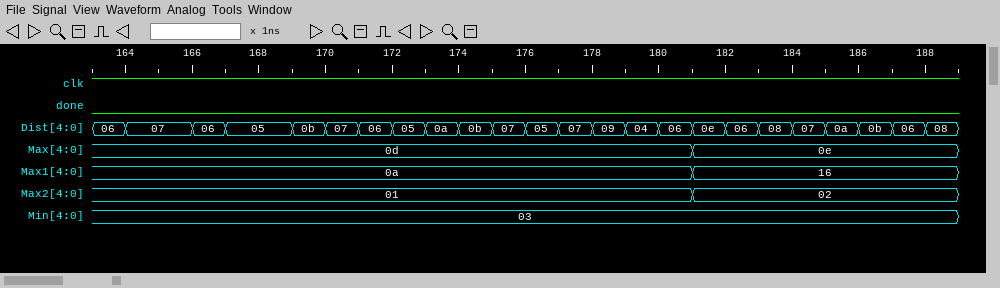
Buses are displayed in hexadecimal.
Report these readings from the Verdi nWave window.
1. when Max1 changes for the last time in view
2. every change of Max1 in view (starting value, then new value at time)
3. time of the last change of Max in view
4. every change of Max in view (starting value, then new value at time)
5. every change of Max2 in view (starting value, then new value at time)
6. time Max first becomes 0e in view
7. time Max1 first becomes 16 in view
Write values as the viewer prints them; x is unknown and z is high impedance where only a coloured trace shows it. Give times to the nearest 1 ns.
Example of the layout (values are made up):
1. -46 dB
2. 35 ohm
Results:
1. 181 ns
2. 0a, 16 at 181 ns
3. 181 ns
4. 0d, 0e at 181 ns
5. 01, 02 at 181 ns
6. 181 ns
7. 181 ns
